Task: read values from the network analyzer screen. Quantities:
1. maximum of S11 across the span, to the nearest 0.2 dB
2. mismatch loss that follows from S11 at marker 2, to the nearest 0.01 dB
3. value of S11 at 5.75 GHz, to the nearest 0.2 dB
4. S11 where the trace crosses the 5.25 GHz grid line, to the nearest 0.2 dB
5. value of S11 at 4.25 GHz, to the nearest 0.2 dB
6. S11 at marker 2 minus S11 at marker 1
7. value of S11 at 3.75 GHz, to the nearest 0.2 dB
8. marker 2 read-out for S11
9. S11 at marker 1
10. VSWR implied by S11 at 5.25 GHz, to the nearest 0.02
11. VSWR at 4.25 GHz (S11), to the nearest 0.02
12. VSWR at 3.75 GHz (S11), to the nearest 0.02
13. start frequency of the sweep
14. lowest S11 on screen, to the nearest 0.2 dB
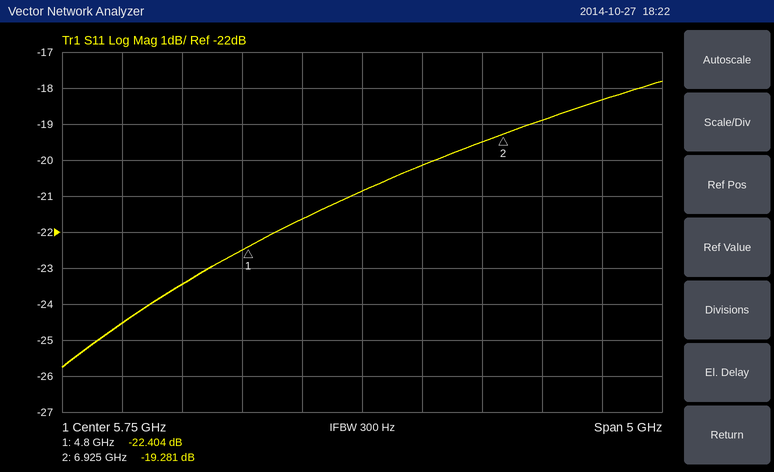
-17.8 dB
0.05 dB
-20.8 dB
-21.6 dB
-23.4 dB
3.123 dB
-24.6 dB
-19.281 dB
-22.404 dB
1.18
1.14
1.12
3.25 GHz
-25.8 dB
